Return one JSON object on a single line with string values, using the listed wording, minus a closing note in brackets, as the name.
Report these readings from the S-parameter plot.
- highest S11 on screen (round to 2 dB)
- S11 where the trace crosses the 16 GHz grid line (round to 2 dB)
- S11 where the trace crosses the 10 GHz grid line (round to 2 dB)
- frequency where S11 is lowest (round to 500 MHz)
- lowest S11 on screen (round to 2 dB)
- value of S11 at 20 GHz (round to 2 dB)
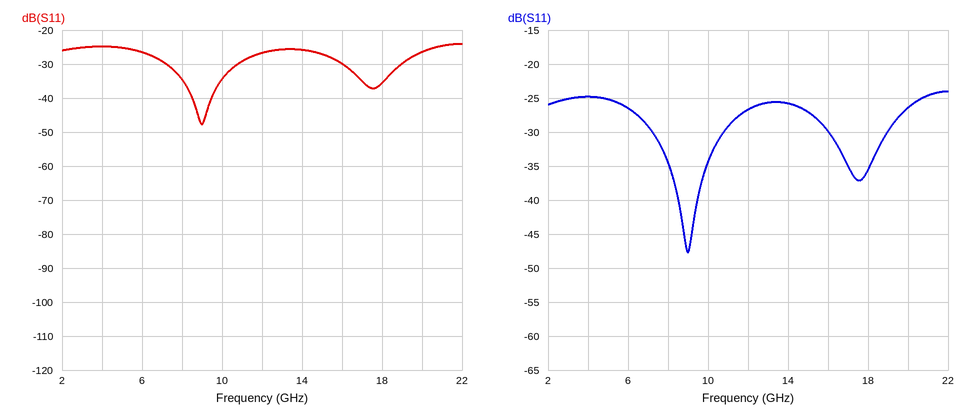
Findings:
{"highest S11 on screen": "-24 dB", "S11 where the trace crosses the 16 GHz grid line": "-30 dB", "S11 where the trace crosses the 10 GHz grid line": "-34 dB", "frequency where S11 is lowest": "9.0 GHz", "lowest S11 on screen": "-48 dB", "value of S11 at 20 GHz": "-26 dB"}
